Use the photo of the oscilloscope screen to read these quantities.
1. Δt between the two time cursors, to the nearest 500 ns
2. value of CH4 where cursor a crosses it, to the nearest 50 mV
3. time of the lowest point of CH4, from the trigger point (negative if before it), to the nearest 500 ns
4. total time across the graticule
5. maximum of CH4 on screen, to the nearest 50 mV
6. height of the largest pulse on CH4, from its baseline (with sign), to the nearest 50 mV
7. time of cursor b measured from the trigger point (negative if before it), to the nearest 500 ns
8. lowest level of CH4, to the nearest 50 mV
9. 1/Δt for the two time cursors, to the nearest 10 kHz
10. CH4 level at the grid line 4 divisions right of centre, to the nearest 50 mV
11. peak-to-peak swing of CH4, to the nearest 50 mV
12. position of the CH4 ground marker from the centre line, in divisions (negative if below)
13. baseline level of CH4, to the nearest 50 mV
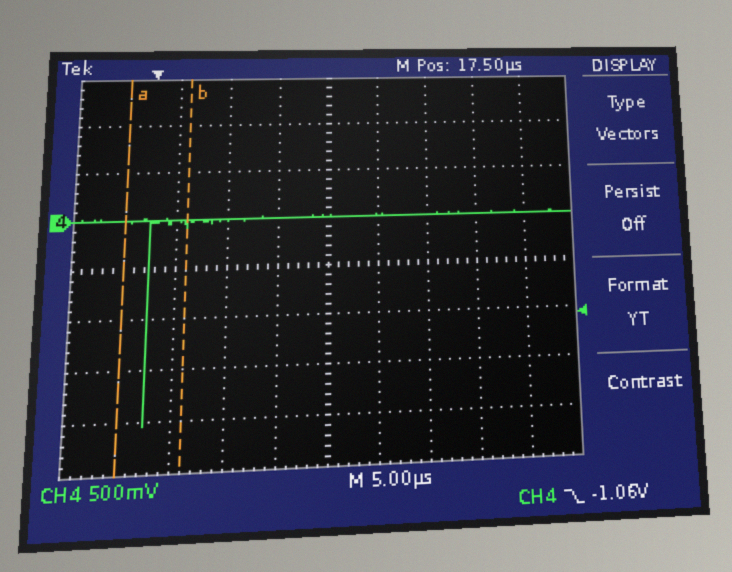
6.0 µs
0 mV
0.0 µs
50 µs
0 mV
-2.05 V
+3.5 µs
-2.05 V
170 kHz
0 mV
2.05 V
+1.0 div
0 mV
